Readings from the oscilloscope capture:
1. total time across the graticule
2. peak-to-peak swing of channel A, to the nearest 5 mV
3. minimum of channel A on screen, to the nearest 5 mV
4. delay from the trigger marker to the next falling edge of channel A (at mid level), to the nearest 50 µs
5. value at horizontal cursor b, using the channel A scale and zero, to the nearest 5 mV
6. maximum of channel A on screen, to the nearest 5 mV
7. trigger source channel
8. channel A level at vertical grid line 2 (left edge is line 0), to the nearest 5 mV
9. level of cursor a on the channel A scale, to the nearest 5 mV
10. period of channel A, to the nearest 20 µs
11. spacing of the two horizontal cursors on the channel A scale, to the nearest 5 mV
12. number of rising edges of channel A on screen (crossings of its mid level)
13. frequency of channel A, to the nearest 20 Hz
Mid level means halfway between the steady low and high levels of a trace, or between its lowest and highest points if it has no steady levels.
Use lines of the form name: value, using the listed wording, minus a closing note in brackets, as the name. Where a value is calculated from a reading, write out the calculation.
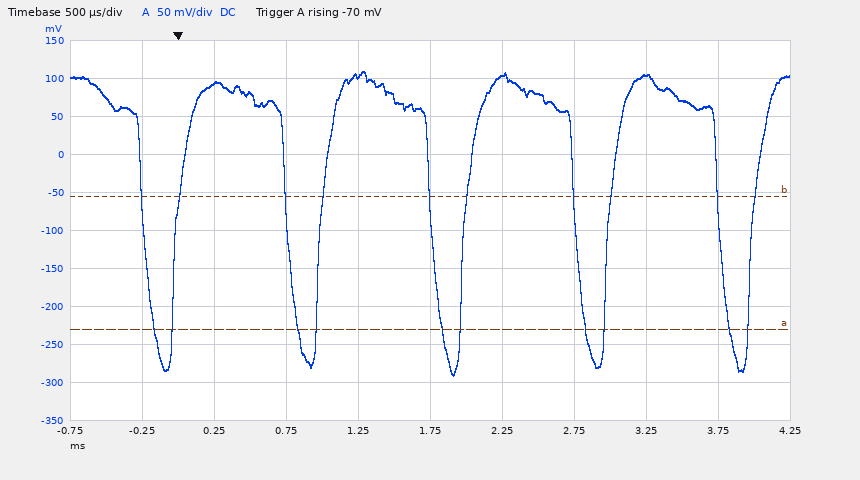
total time across the graticule: 5 ms
peak-to-peak swing of channel A, to the nearest 5 mV: 110 mV − (-290 mV) = 400 mV
minimum of channel A on screen, to the nearest 5 mV: -290 mV
delay from the trigger marker to the next falling edge of channel A (at mid level), to the nearest 50 µs: 750 µs
value at horizontal cursor b, using the channel A scale and zero, to the nearest 5 mV: -55 mV
maximum of channel A on screen, to the nearest 5 mV: 110 mV
trigger source channel: channel A
channel A level at vertical grid line 2 (left edge is line 0), to the nearest 5 mV: 95 mV
level of cursor a on the channel A scale, to the nearest 5 mV: -230 mV
period of channel A, to the nearest 20 µs: 1.00 ms
spacing of the two horizontal cursors on the channel A scale, to the nearest 5 mV: 175 mV
number of rising edges of channel A on screen: 5
frequency of channel A, to the nearest 20 Hz: 1 / 1.00 ms ≈ 1.00 kHz
